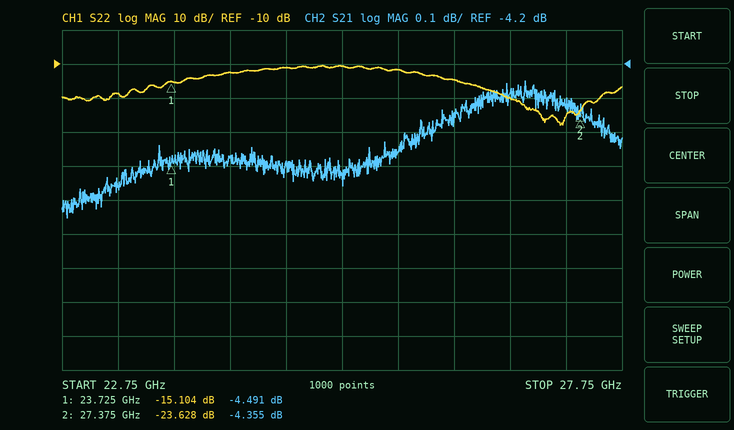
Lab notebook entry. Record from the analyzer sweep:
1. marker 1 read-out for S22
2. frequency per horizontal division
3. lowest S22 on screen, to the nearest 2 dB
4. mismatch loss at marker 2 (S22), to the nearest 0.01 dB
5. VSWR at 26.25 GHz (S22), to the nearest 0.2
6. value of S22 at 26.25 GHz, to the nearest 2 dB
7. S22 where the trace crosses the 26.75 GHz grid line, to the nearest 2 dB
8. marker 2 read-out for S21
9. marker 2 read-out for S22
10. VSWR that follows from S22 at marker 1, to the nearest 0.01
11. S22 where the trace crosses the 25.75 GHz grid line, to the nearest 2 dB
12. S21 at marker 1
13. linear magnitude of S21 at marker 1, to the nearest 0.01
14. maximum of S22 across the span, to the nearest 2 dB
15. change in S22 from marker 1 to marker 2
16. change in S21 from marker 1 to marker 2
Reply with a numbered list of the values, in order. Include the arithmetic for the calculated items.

1. -15.104 dB
2. 500 MHz
3. -28 dB
4. −10 log10(1 − 10^(-23.628/10)) ≈ 0.02 dB
5. |Γ| = 10^(-14/20) = 0.1995; VSWR = (1 + 0.1995)/(1 − 0.1995) ≈ 1.50, so 1.4 to the nearest 0.2
6. -14 dB
7. -20 dB
8. -4.355 dB
9. -23.628 dB
10. (1 + 0.1757)/(1 − 0.1757) ≈ 1.43
11. -12 dB
12. -4.491 dB
13. 10^(-4.491/20) ≈ 0.60
14. -10 dB
15. -23.628 − (-15.104) = -8.524 dB
16. -4.355 − (-4.491) = 0.136 dB
